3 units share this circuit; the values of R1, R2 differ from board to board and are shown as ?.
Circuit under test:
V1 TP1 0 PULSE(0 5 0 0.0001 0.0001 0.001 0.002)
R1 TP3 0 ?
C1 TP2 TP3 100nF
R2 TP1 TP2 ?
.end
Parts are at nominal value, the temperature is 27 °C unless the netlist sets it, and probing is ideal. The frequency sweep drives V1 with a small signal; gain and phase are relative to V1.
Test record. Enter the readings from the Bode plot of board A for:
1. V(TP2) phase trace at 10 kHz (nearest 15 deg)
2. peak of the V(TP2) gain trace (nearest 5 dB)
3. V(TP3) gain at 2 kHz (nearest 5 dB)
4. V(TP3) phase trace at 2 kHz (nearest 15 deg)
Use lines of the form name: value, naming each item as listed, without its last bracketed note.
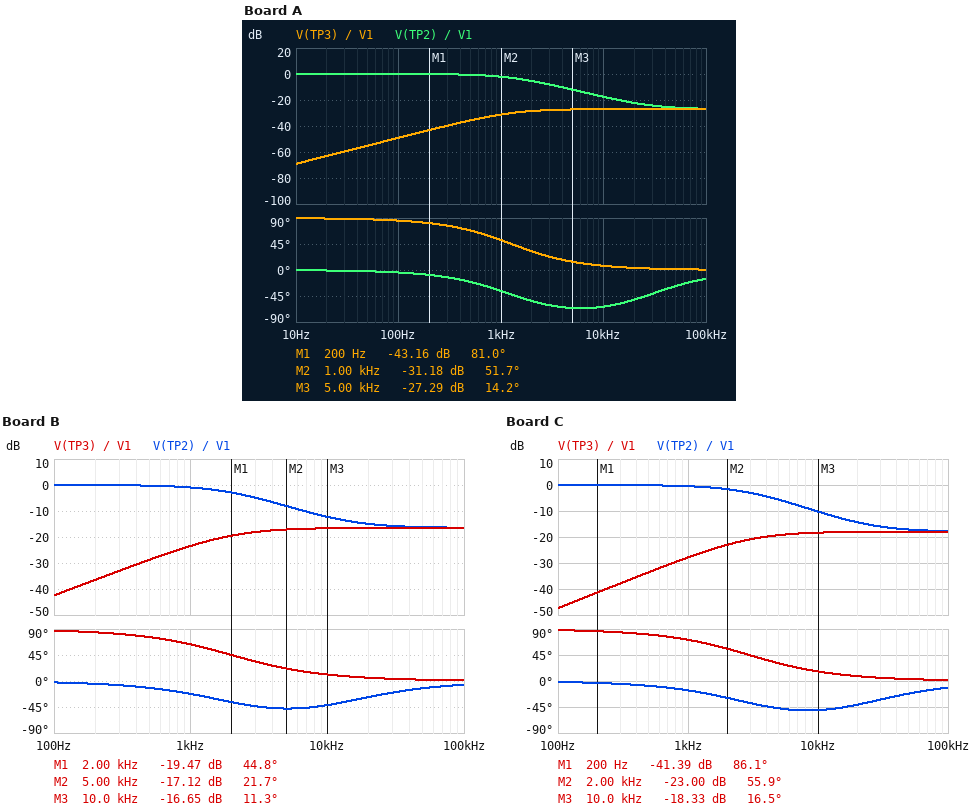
V(TP2) phase trace at 10 kHz: -60 deg
peak of the V(TP2) gain trace: 0 dB
V(TP3) gain at 2 kHz: -30 dB
V(TP3) phase trace at 2 kHz: 30 deg
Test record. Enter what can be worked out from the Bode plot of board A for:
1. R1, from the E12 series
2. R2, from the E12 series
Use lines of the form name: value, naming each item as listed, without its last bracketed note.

R1, from the E12 series: 56 Ω
R2, from the E12 series: 1.2 kΩ
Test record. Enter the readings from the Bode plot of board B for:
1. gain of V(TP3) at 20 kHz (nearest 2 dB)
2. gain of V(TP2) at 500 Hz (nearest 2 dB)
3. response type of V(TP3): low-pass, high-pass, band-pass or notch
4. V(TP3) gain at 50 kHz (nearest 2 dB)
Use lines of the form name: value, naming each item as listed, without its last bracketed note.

gain of V(TP3) at 20 kHz: -16 dB
gain of V(TP2) at 500 Hz: 0 dB
response type of V(TP3): low-pass, high-pass, band-pass or notch: high-pass
V(TP3) gain at 50 kHz: -16 dB
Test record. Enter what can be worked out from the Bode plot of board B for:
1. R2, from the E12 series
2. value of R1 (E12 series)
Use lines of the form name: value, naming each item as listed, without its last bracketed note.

R2, from the E12 series: 680 Ω
value of R1: 120 Ω
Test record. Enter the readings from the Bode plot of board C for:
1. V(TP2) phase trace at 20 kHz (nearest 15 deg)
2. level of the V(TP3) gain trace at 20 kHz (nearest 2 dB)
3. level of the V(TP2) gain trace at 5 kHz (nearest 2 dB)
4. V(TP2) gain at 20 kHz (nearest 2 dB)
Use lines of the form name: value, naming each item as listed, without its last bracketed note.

V(TP2) phase trace at 20 kHz: -45 deg
level of the V(TP3) gain trace at 20 kHz: -18 dB
level of the V(TP2) gain trace at 5 kHz: -6 dB
V(TP2) gain at 20 kHz: -14 dB
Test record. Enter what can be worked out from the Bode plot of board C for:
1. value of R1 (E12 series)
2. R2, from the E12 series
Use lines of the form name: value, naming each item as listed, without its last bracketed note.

value of R1: 68 Ω
R2, from the E12 series: 470 Ω
